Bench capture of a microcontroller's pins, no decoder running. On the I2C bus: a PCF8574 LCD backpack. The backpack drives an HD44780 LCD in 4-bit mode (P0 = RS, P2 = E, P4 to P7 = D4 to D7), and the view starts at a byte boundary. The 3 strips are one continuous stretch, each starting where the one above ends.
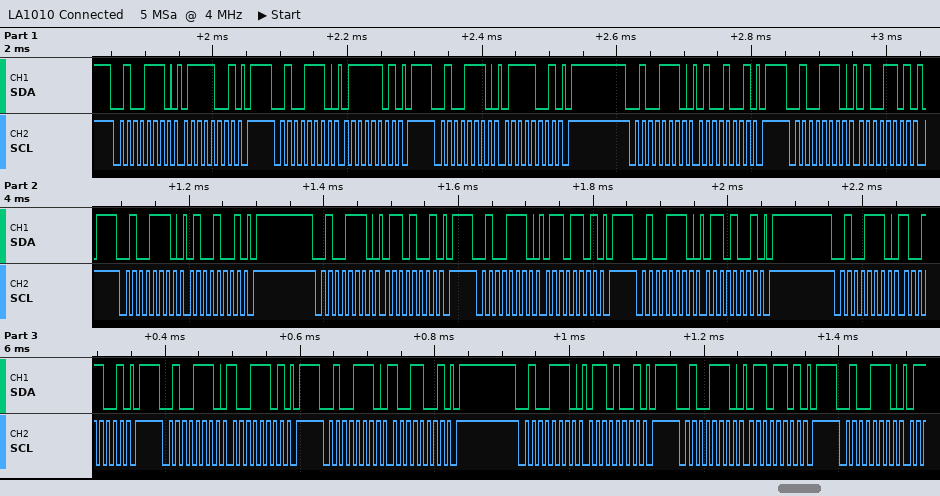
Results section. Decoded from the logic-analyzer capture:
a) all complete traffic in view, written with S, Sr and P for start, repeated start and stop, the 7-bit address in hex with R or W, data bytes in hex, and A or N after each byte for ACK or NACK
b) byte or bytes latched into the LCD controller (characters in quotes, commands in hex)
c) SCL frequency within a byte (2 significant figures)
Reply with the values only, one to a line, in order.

S 27W A 79 A P S 27W A 7D A P S 27W A 79 A P S 27W A 49 A P S 27W A 4D A P S 27W A 49 A P S 27W A 69 A P S 27W A 6D A P S 27W A 69 A P S 27W A 99 A P S 27W A 9D A P S 27W A 99 A P S 27W A 69 A P S 27W A 6D A P S 27W A
't' 'i'
100 kHz
